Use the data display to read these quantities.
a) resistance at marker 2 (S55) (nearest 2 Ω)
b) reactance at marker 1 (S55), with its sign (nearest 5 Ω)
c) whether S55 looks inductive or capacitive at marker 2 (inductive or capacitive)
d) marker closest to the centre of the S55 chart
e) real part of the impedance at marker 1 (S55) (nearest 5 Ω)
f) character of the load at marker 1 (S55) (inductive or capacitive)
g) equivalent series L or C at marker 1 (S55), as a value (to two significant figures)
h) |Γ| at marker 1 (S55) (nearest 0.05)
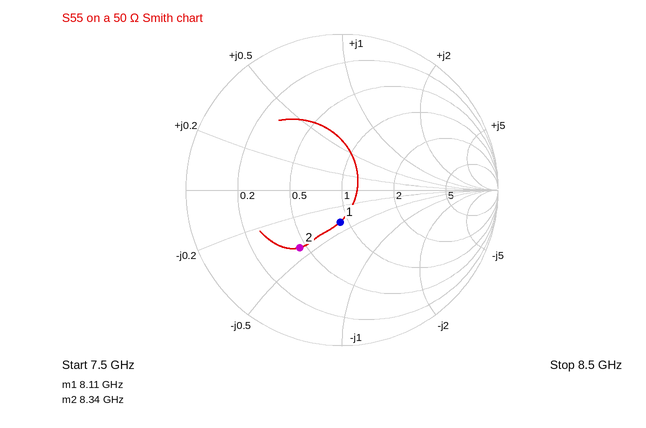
22 Ω
-20 Ω
capacitive
marker 1
45 Ω
capacitive
1.0 pF
0.20
